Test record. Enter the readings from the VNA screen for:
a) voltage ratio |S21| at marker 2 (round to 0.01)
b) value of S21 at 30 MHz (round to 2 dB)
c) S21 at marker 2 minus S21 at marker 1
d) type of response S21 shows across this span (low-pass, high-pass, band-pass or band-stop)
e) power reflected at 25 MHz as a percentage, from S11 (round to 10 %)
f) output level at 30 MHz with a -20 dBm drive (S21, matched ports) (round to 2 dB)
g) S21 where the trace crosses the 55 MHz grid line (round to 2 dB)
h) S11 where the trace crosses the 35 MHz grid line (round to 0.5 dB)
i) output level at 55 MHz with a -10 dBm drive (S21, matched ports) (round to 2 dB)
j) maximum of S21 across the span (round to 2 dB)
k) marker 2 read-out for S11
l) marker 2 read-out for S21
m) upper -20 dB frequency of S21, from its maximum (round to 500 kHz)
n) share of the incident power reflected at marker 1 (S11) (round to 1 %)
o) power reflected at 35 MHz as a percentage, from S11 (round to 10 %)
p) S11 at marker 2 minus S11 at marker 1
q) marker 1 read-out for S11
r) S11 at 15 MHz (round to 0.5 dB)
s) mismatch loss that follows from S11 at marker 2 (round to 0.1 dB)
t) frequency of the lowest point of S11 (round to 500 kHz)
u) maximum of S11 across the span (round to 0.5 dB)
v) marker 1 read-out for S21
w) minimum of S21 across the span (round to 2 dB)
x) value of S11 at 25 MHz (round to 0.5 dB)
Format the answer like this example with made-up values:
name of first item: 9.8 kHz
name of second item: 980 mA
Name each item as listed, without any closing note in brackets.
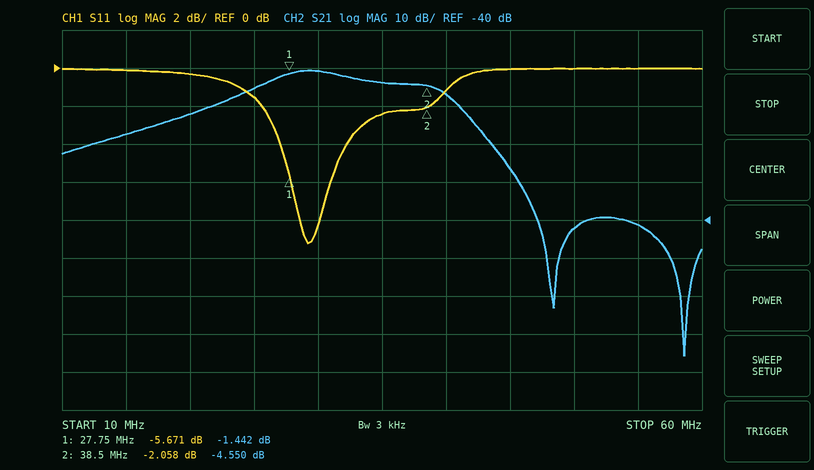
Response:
voltage ratio |S21| at marker 2: 0.59
value of S21 at 30 MHz: 0 dB
S21 at marker 2 minus S21 at marker 1: -3.108 dB
type of response S21 shows across this span: band-pass
power reflected at 25 MHz as a percentage, from S11: 70 %
output level at 30 MHz with a -20 dBm drive (S21, matched ports): -20 dBm
S21 where the trace crosses the 55 MHz grid line: -42 dB
S11 where the trace crosses the 35 MHz grid line: -2.5 dB
output level at 55 MHz with a -10 dBm drive (S21, matched ports): -52 dBm
maximum of S21 across the span: 0 dB
marker 2 read-out for S11: -2.058 dB
marker 2 read-out for S21: -4.550 dB
upper -20 dB frequency of S21, from its maximum: 43.5 MHz
share of the incident power reflected at marker 1 (S11): 27 %
power reflected at 35 MHz as a percentage, from S11: 60 %
S11 at marker 2 minus S11 at marker 1: 3.613 dB
marker 1 read-out for S11: -5.671 dB
S11 at 15 MHz: 0.0 dB
mismatch loss that follows from S11 at marker 2: 4.2 dB
frequency of the lowest point of S11: 29.0 MHz
maximum of S11 across the span: 0.0 dB
marker 1 read-out for S21: -1.442 dB
minimum of S21 across the span: -76 dB
value of S11 at 25 MHz: -1.5 dB
